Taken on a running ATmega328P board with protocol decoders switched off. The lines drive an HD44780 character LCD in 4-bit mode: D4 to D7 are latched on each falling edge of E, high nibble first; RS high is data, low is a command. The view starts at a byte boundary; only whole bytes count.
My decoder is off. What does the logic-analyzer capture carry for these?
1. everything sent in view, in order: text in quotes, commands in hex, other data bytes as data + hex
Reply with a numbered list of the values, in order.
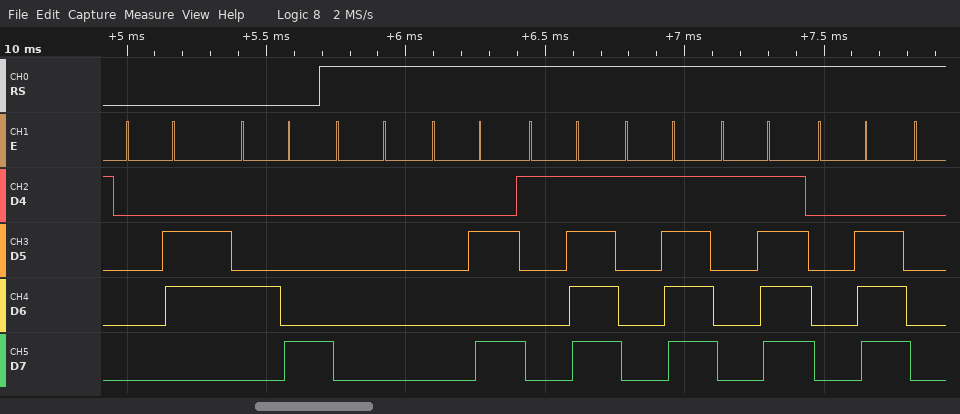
1. 0x06 0x48 data 00 0A 1F 1F 1F 0E
